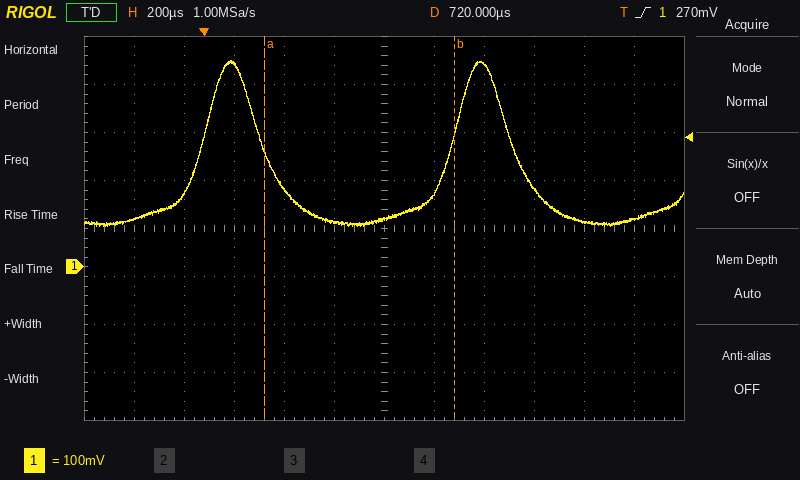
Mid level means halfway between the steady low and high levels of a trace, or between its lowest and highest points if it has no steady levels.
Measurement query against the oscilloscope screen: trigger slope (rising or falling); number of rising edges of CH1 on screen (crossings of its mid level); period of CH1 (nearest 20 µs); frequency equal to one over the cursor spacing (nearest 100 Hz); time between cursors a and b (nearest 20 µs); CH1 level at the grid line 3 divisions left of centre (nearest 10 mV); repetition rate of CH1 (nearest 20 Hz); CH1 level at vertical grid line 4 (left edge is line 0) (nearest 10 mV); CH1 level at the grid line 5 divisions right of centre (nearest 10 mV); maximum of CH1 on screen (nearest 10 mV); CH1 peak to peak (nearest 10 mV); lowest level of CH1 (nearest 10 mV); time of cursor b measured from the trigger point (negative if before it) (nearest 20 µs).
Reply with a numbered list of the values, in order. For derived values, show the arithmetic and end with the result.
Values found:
1. rising
2. 2
3. 1.00 ms
4. 1 / 760 µs ≈ 1.3 kHz
5. 760 µs
6. 420 mV
7. 1 / 1.00 ms ≈ 1.00 kHz
8. 160 mV
9. 100 mV
10. 430 mV
11. 430 mV − (80 mV) = 350 mV
12. 80 mV
13. +1.00 ms
